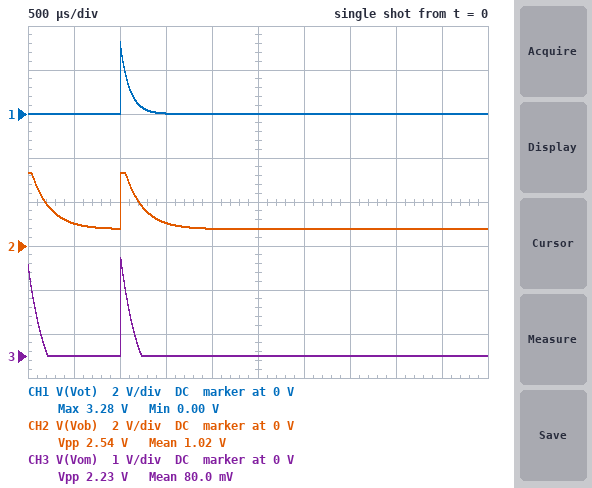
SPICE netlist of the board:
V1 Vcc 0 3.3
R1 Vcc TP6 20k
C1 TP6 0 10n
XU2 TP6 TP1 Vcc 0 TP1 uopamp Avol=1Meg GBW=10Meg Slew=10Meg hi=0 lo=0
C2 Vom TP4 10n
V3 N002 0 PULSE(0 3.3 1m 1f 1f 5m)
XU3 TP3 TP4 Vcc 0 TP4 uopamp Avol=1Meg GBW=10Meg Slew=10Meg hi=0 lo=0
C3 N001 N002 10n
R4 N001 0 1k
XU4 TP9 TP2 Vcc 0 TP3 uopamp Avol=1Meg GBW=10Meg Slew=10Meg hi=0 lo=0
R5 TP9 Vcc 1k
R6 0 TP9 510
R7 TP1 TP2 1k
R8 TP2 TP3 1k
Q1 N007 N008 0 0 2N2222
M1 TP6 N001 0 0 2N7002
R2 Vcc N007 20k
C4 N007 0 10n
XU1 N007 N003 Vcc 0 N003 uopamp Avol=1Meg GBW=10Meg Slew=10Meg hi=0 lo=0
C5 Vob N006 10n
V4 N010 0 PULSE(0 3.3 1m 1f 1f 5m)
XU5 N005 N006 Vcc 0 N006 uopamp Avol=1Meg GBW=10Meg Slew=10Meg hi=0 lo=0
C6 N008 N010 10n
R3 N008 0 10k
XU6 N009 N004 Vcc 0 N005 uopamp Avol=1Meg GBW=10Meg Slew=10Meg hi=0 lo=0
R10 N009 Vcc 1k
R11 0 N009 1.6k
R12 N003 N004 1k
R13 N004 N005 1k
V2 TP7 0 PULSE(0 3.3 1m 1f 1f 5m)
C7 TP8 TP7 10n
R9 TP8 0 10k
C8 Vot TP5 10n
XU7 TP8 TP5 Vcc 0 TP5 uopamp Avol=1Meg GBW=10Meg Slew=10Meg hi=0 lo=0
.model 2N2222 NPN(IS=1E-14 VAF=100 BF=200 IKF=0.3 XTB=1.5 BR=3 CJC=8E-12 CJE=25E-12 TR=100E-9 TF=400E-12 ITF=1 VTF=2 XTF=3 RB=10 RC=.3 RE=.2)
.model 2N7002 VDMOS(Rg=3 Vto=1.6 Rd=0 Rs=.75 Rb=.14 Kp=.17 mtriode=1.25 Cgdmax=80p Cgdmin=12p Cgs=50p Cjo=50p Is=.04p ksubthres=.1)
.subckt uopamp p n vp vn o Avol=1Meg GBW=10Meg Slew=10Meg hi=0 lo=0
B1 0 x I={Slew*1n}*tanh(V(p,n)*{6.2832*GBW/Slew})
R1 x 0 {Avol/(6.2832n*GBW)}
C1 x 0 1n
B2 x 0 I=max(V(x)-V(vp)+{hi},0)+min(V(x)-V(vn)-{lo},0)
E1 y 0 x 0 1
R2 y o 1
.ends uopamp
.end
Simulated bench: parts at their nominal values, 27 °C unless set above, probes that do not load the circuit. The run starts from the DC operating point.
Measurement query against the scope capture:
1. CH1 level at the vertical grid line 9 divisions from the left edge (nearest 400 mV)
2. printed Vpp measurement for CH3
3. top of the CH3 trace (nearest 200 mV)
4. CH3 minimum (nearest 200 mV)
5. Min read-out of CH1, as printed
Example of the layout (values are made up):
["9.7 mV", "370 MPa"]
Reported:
["0 V", "2.23 V", "2.2 V", "0 V", "0.00 V"]
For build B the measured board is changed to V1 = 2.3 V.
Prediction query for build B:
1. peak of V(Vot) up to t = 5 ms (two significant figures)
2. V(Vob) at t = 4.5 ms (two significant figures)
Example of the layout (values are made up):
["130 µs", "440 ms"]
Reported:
["2.3 V", "530 mV"]
